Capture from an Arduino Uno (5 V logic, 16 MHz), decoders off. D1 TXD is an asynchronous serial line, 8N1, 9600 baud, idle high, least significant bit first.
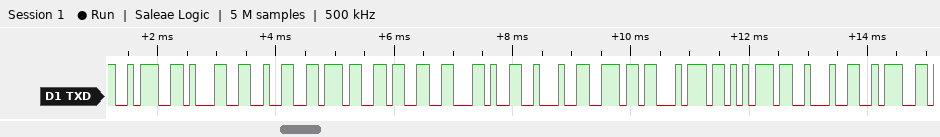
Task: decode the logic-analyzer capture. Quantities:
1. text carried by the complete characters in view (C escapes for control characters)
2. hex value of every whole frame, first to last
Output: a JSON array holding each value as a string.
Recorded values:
["\":1273,\\\"ntu\\\":\"", "0x3A 0x31 0x32 0x37 0x33 0x2C 0x22 0x6E 0x74 0x75 0x22 0x3A"]
